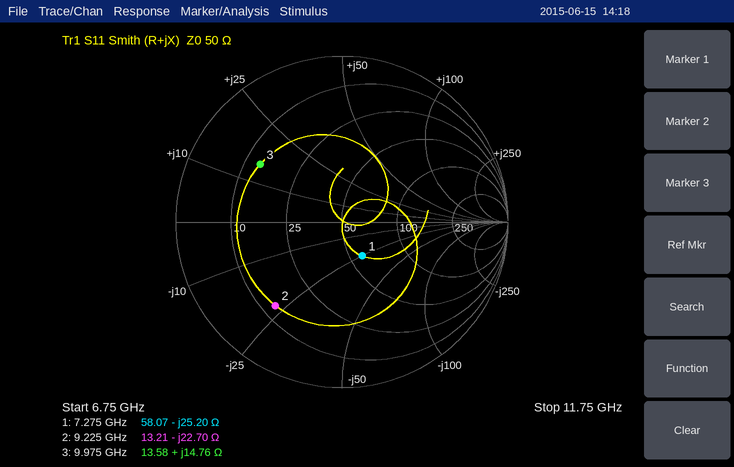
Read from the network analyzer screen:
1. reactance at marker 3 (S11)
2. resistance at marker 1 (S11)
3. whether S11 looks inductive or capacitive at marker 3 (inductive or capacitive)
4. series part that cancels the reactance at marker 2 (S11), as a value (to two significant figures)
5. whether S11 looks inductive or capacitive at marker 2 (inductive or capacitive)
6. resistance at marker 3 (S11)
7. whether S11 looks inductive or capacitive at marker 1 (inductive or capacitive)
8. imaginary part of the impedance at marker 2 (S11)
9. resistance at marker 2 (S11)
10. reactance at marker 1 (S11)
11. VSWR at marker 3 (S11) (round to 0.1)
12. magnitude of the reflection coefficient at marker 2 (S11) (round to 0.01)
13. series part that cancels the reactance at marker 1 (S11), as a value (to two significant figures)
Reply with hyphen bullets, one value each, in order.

- +14.76 Ω
- 58.07 Ω
- inductive
- 390 pH
- capacitive
- 13.58 Ω
- capacitive
- -22.70 Ω
- 13.21 Ω
- -25.20 Ω
- 4.0
- 0.64
- 550 pH
